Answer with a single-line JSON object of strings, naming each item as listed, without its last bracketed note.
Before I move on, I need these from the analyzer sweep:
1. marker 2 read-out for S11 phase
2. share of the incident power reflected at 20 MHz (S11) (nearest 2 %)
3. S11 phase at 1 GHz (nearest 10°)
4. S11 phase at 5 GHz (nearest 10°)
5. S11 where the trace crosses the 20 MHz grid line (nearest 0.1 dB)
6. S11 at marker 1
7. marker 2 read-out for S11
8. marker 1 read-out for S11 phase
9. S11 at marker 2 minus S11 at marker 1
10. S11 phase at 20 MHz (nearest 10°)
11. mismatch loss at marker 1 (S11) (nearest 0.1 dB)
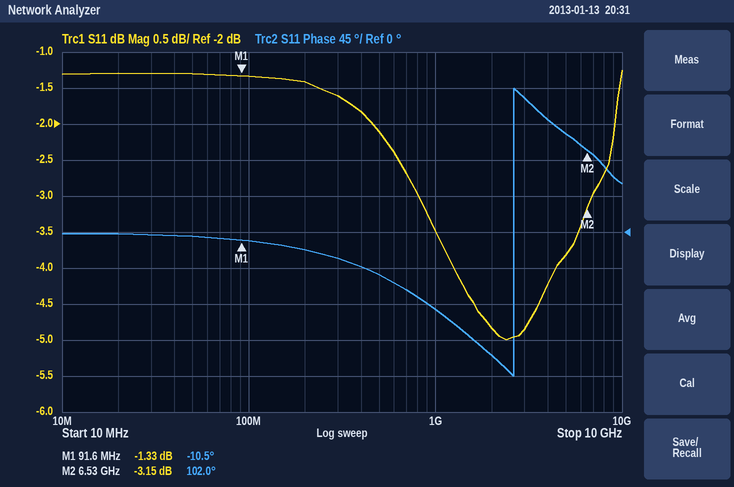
{"marker 2 read-out for S11 phase": "102.0°", "share of the incident power reflected at 20 MHz (S11)": "74 %", "S11 phase at 1 GHz": "-100°", "S11 phase at 5 GHz": "120°", "S11 where the trace crosses the 20 MHz grid line": "-1.3 dB", "S11 at marker 1": "-1.33 dB", "marker 2 read-out for S11": "-3.15 dB", "marker 1 read-out for S11 phase": "-10.5°", "S11 at marker 2 minus S11 at marker 1": "-1.82 dB", "S11 phase at 20 MHz": "0°", "mismatch loss at marker 1 (S11)": "5.8 dB"}
